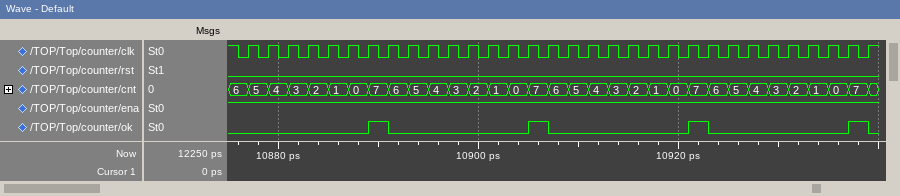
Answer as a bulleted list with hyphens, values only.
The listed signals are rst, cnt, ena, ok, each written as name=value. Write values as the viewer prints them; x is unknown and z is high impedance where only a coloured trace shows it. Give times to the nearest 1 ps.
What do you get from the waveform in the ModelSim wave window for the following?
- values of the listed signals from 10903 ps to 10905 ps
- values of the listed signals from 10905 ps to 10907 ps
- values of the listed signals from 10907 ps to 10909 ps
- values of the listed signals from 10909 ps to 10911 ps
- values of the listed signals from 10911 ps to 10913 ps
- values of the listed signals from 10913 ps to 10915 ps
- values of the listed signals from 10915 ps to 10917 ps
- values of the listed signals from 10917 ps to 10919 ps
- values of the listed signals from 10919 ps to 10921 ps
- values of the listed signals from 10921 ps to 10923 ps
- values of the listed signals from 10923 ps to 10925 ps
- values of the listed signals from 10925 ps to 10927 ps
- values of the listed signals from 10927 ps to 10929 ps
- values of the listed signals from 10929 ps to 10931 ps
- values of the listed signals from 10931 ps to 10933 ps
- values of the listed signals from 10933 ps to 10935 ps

- rst=0, cnt=0, ena=1, ok=0
- rst=0, cnt=7, ena=1, ok=1
- rst=0, cnt=6, ena=1, ok=0
- rst=0, cnt=5, ena=1, ok=0
- rst=0, cnt=4, ena=1, ok=0
- rst=0, cnt=3, ena=1, ok=0
- rst=0, cnt=2, ena=1, ok=0
- rst=0, cnt=1, ena=1, ok=0
- rst=0, cnt=0, ena=1, ok=0
- rst=0, cnt=7, ena=1, ok=1
- rst=0, cnt=6, ena=1, ok=0
- rst=0, cnt=5, ena=1, ok=0
- rst=0, cnt=4, ena=1, ok=0
- rst=0, cnt=3, ena=1, ok=0
- rst=0, cnt=2, ena=1, ok=0
- rst=0, cnt=1, ena=1, ok=0
